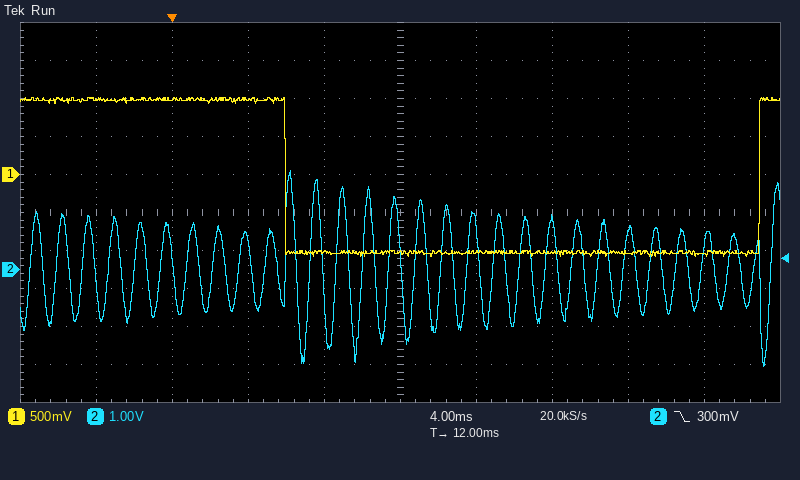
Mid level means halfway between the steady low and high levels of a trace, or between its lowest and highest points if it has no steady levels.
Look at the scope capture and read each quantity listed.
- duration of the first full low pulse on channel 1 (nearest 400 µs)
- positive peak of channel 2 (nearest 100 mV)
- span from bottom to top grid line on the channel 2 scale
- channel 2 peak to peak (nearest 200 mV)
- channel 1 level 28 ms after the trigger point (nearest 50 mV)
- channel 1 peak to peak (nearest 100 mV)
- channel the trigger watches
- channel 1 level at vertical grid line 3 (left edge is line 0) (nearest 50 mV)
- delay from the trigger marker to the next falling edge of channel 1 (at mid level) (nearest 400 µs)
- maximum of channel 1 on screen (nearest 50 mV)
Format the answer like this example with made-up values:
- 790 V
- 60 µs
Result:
- 24.8 ms
- 2.6 V
- 10 V
- 5.2 V
- -1.05 V
- 2.10 V
- channel 2
- 1.00 V
- 6.0 ms
- 1.00 V
